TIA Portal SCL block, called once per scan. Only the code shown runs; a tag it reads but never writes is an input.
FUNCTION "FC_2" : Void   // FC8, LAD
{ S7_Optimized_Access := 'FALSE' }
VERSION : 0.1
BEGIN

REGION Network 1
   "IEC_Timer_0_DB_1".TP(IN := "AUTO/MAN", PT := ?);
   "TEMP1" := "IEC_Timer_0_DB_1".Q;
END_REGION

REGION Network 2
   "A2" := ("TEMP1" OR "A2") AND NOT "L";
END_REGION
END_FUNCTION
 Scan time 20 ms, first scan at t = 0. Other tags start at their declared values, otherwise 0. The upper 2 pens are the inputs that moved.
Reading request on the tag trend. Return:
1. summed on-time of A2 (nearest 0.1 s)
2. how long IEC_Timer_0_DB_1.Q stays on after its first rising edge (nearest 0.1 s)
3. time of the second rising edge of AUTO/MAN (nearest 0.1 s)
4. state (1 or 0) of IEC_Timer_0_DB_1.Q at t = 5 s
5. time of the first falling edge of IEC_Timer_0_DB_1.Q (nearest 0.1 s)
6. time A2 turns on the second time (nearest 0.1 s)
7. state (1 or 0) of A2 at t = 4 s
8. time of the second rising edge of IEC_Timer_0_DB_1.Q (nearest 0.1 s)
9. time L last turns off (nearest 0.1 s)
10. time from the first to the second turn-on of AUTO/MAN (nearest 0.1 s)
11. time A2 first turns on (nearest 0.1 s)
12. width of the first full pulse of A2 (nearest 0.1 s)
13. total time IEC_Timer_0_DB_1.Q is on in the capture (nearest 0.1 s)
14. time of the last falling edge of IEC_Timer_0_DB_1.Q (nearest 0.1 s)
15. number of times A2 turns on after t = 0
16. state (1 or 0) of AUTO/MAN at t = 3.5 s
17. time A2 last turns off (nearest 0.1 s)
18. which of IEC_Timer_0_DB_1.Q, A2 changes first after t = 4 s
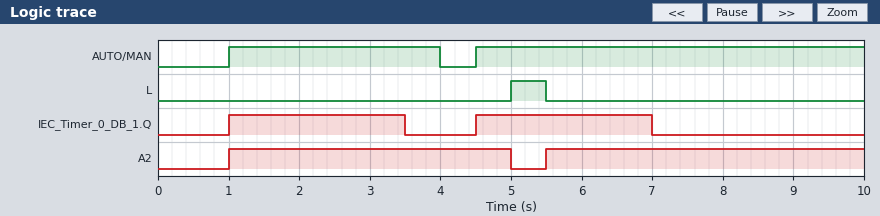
8.5 s
2.5 s
4.5 s
1
3.5 s
5.5 s
1
4.5 s
5.5 s
3.5 s
1.0 s
4.0 s
5.0 s
7.0 s
2
1
5.0 s
IEC_Timer_0_DB_1.Q
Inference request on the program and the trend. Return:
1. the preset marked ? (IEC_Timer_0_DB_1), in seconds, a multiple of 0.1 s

2.5 s
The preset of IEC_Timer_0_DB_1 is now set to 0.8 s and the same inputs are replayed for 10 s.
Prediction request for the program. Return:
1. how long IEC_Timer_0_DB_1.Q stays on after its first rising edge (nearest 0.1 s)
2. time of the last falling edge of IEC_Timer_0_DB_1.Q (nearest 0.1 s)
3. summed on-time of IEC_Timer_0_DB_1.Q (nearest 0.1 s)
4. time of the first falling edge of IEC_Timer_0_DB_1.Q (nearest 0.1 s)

0.8 s
5.3 s
1.6 s
1.8 s
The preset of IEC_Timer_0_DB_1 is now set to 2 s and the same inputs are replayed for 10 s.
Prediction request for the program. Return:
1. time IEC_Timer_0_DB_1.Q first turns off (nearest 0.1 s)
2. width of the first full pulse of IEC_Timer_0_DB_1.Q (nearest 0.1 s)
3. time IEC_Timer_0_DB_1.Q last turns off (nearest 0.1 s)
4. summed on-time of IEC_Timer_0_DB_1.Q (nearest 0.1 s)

3.0 s
2.0 s
6.5 s
4.0 s
